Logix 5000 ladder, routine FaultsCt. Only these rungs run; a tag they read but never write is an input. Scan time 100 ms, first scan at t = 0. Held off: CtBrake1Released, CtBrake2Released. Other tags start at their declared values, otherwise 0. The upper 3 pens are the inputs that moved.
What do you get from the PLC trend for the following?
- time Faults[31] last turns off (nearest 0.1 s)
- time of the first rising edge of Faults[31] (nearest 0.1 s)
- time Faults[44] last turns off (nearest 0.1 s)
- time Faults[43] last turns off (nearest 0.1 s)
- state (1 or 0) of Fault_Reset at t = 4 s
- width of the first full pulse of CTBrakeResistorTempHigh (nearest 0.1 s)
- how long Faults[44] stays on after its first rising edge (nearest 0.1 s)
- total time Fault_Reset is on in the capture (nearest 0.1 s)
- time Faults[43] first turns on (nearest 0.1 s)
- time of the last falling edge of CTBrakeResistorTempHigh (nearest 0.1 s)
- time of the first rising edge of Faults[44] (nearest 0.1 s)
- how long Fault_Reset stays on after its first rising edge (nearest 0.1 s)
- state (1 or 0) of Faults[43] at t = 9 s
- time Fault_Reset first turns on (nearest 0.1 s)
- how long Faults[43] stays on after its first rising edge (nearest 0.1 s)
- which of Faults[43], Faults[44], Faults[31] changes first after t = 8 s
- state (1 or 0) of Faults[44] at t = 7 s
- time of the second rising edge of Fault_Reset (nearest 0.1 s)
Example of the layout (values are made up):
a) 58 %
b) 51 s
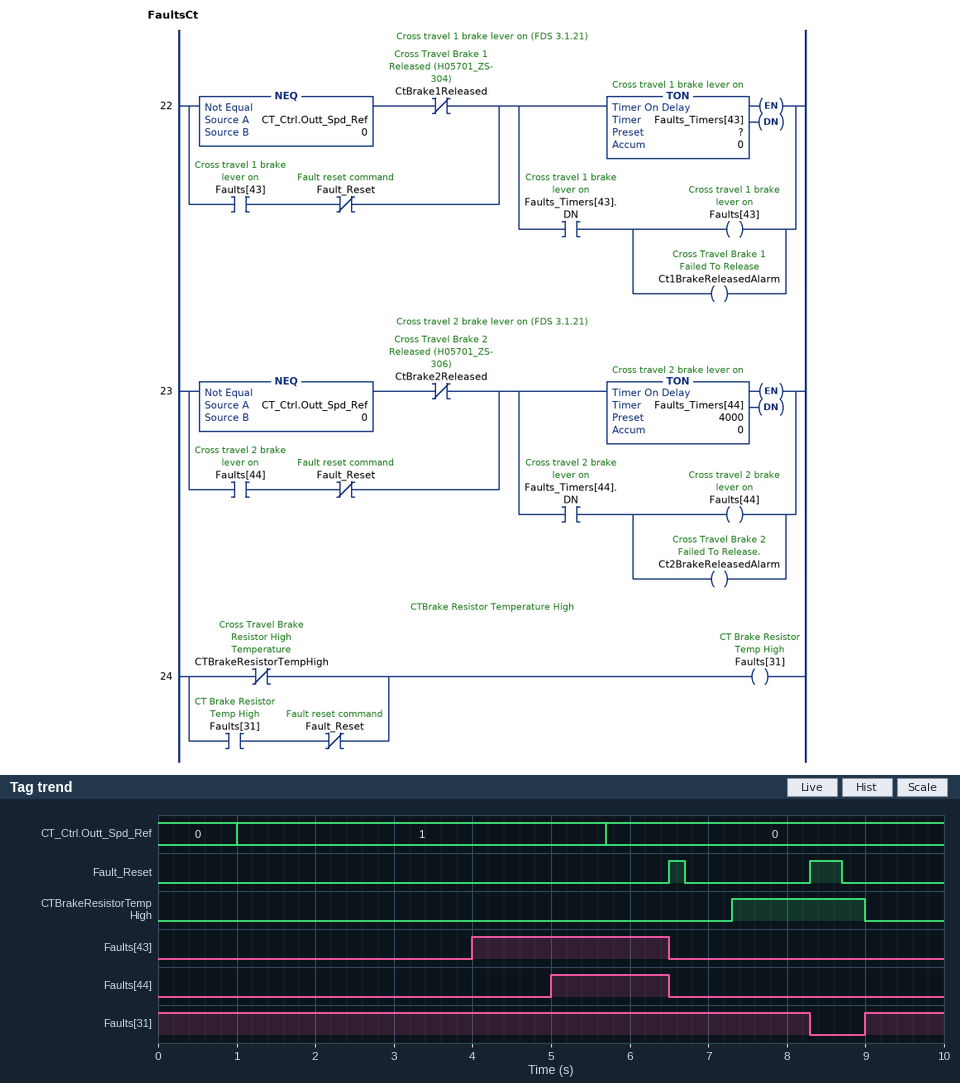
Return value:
a) 8.3 s
b) 9.0 s
c) 6.5 s
d) 6.5 s
e) 0
f) 1.7 s
g) 1.5 s
h) 0.6 s
i) 4.0 s
j) 9.0 s
k) 5.0 s
l) 0.2 s
m) 0
n) 6.5 s
o) 2.5 s
p) Faults[31]
q) 0
r) 8.3 s
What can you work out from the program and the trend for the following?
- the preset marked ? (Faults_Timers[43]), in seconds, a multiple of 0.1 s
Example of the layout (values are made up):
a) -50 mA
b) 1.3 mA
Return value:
a) 3.0 s
